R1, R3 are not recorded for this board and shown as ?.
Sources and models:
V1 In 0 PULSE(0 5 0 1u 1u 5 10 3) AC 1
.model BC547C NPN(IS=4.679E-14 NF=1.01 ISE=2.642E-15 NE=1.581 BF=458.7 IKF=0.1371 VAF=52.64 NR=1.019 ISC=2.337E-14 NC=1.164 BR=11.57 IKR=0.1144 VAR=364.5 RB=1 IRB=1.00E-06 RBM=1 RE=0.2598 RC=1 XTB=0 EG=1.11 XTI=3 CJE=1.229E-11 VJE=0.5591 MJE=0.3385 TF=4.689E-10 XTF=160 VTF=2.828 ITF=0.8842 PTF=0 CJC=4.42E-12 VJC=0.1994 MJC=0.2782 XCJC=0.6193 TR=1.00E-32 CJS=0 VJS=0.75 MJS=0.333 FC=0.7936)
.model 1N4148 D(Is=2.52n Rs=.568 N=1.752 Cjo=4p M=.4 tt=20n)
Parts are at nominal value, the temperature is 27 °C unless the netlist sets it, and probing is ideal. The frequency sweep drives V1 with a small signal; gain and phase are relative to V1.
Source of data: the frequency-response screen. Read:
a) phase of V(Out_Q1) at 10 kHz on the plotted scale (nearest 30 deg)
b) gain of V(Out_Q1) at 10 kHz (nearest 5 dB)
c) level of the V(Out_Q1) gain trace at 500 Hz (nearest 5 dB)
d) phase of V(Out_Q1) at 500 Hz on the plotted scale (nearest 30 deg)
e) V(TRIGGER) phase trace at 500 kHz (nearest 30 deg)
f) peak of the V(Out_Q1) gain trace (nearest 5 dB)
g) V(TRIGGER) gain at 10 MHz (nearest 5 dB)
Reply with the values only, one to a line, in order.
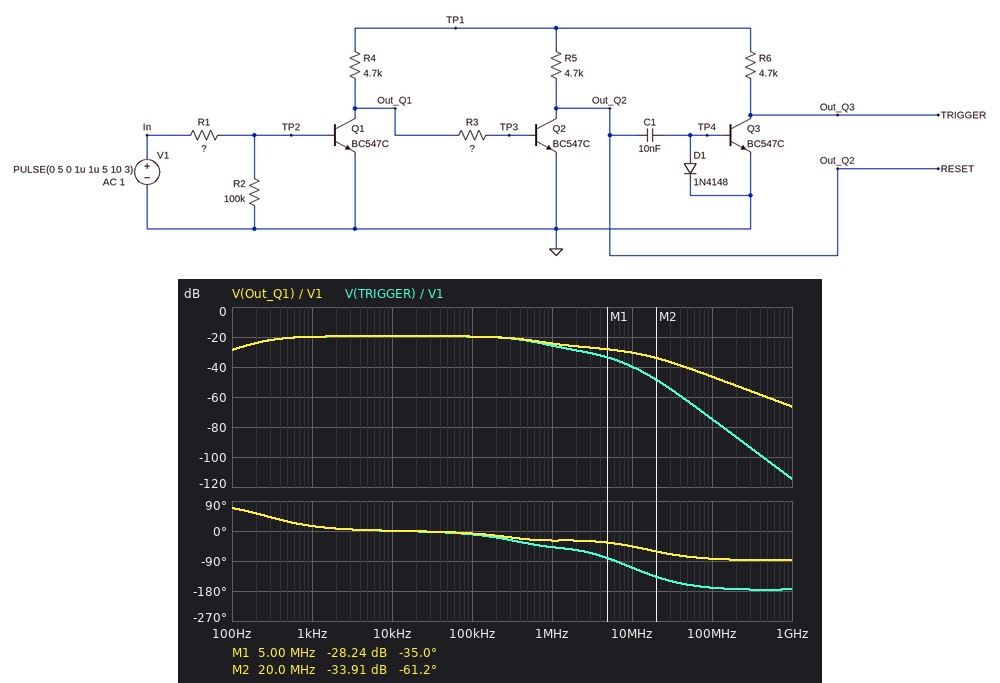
0 deg
-20 dB
-20 dB
30 deg
-30 deg
-20 dB
-40 dB
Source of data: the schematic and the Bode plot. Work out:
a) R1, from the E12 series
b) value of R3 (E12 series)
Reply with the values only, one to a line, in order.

27 kΩ
12 kΩ
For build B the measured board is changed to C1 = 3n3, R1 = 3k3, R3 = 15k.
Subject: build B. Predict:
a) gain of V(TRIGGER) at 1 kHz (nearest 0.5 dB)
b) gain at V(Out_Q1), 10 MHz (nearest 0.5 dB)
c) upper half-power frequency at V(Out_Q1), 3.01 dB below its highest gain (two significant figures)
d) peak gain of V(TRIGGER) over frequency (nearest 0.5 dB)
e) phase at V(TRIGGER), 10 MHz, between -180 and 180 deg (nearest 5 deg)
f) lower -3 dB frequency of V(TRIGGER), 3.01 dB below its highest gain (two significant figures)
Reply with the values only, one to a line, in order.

-18.0 dB
-12.5 dB
15 MHz
-15.5 dB
-95 deg
720 Hz
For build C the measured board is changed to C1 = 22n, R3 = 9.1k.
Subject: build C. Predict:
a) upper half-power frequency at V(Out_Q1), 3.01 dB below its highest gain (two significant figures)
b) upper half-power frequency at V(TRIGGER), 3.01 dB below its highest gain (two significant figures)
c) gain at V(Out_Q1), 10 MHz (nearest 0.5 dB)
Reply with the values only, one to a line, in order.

560 kHz
480 kHz
-31.0 dB
